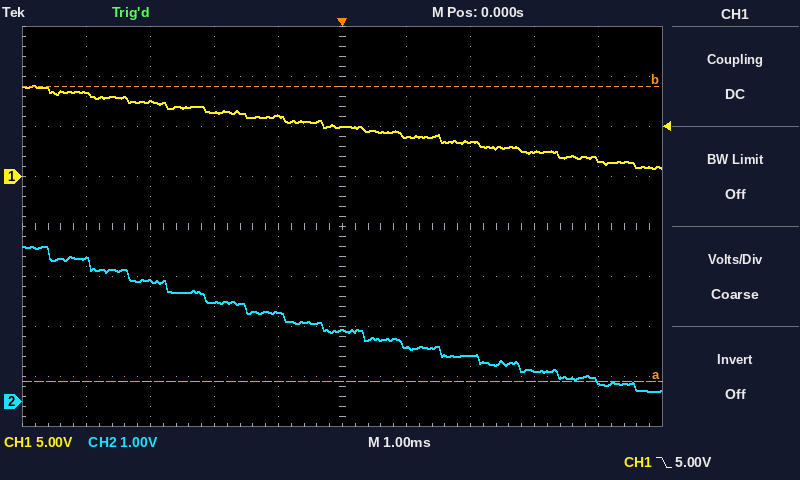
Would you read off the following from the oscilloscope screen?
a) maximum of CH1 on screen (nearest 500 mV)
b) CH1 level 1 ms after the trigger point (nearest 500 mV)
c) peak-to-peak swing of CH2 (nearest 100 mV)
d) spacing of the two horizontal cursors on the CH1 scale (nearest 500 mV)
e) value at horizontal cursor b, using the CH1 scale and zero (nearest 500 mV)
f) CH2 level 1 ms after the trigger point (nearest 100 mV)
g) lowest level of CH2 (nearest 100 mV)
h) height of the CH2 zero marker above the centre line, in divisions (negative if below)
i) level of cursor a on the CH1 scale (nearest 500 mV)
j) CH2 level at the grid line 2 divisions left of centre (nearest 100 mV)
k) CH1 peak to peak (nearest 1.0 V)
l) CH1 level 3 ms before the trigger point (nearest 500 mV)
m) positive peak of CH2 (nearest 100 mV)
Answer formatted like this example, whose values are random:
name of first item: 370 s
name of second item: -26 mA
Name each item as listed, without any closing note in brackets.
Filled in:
maximum of CH1 on screen: 9.0 V
CH1 level 1 ms after the trigger point: 4.0 V
peak-to-peak swing of CH2: 2.9 V
spacing of the two horizontal cursors on the CH1 scale: 29.5 V
value at horizontal cursor b, using the CH1 scale and zero: 9.0 V
CH2 level 1 ms after the trigger point: 1.1 V
lowest level of CH2: 200 mV
height of the CH2 zero marker above the centre line, in divisions: -3.5 div
level of cursor a on the CH1 scale: -20.5 V
CH2 level at the grid line 2 divisions left of centre: 2.0 V
CH1 peak to peak: 8.0 V
CH1 level 3 ms before the trigger point: 7.5 V
positive peak of CH2: 3.1 V
